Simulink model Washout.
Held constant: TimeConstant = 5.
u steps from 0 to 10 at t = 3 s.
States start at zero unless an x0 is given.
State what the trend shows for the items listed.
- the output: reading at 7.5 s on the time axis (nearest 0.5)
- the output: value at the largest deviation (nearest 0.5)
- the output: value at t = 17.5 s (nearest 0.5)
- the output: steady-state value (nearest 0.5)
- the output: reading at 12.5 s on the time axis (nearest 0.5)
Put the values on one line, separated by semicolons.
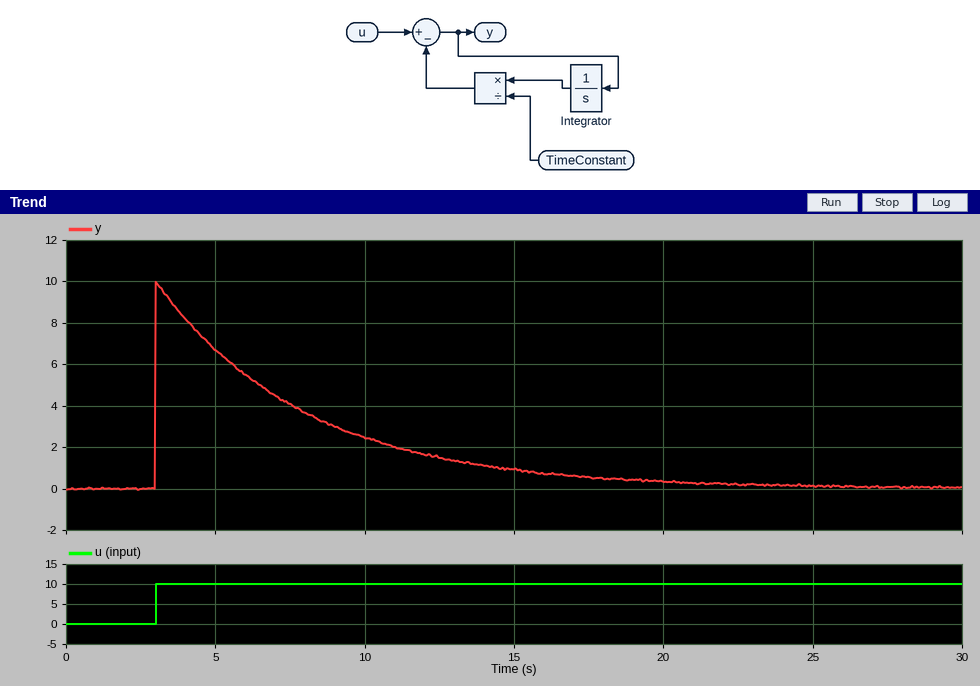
4.0; 10.0; 0.5; 0.0; 1.5
